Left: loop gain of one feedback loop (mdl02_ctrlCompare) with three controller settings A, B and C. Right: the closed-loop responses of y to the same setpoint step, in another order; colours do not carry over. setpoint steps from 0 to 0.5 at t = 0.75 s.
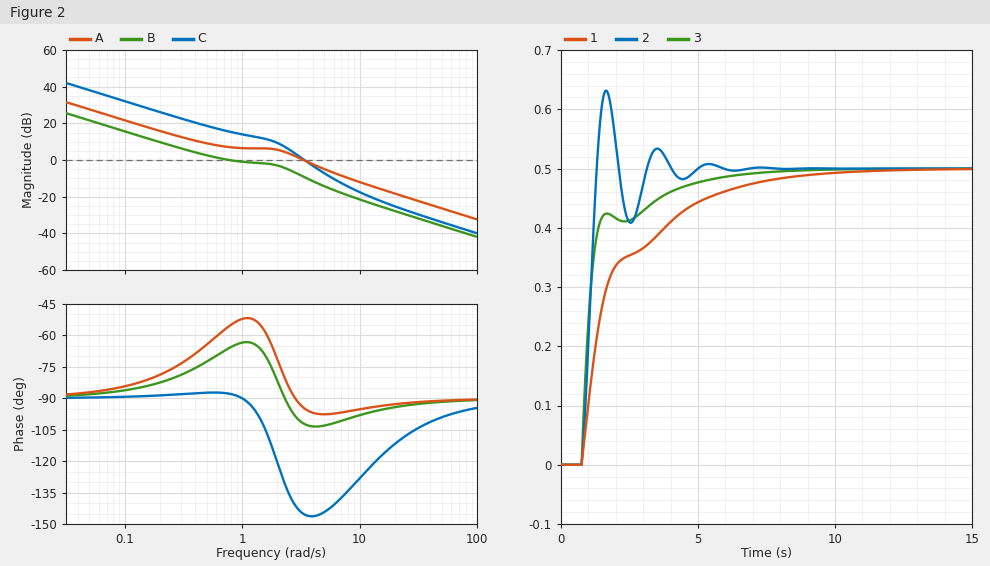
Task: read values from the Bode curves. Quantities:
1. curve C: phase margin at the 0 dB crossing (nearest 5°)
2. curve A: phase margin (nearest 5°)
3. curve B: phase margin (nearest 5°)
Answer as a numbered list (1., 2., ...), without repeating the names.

1. 35°
2. 85°
3. 115°
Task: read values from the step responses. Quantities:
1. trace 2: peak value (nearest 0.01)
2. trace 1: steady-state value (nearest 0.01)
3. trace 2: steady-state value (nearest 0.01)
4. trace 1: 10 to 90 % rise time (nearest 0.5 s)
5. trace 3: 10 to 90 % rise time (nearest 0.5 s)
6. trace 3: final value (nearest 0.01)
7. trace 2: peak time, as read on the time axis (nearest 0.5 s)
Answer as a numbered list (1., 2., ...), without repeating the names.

1. 0.63
2. 0.50
3. 0.50
4. 4.5 s
5. 3.0 s
6. 0.50
7. 1.5 s
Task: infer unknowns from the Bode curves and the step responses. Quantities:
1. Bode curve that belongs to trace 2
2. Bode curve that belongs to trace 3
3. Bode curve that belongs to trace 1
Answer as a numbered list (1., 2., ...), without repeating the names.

1. C
2. A
3. B
